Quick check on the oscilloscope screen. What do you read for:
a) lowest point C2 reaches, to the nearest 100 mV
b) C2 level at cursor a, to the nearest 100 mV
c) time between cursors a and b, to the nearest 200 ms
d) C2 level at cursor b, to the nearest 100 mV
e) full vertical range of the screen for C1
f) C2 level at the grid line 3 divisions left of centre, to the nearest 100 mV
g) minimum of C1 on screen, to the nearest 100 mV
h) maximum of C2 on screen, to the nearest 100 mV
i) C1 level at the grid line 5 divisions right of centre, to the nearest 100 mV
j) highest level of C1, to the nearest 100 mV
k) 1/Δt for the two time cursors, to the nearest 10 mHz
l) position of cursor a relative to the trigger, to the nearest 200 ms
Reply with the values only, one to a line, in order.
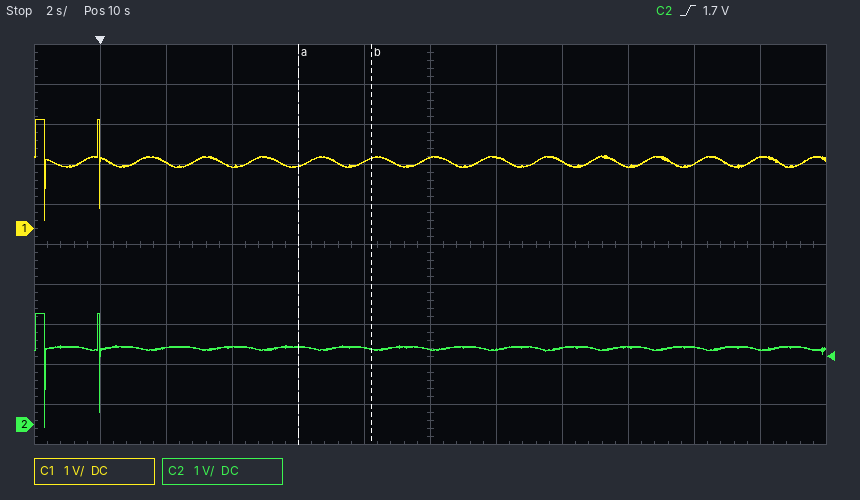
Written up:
-100 mV
1.9 V
2.2 s
1.9 V
10 V
1.9 V
200 mV
2.8 V
1.8 V
2.7 V
450 mHz
+6.0 s
